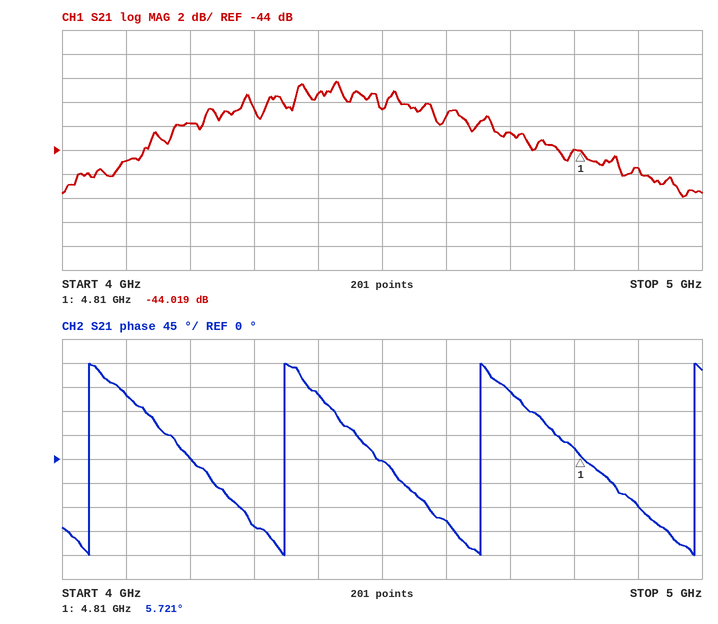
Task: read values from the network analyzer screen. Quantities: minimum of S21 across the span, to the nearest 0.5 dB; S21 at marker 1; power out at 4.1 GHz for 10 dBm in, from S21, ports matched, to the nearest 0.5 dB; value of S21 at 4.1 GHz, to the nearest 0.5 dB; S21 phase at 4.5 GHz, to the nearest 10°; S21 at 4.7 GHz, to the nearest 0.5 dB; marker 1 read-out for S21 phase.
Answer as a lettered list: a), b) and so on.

a) -48.0 dB
b) -44.019 dB
c) -35.0 dBm
d) -45.0 dB
e) 0°
f) -42.5 dB
g) 5.721°
